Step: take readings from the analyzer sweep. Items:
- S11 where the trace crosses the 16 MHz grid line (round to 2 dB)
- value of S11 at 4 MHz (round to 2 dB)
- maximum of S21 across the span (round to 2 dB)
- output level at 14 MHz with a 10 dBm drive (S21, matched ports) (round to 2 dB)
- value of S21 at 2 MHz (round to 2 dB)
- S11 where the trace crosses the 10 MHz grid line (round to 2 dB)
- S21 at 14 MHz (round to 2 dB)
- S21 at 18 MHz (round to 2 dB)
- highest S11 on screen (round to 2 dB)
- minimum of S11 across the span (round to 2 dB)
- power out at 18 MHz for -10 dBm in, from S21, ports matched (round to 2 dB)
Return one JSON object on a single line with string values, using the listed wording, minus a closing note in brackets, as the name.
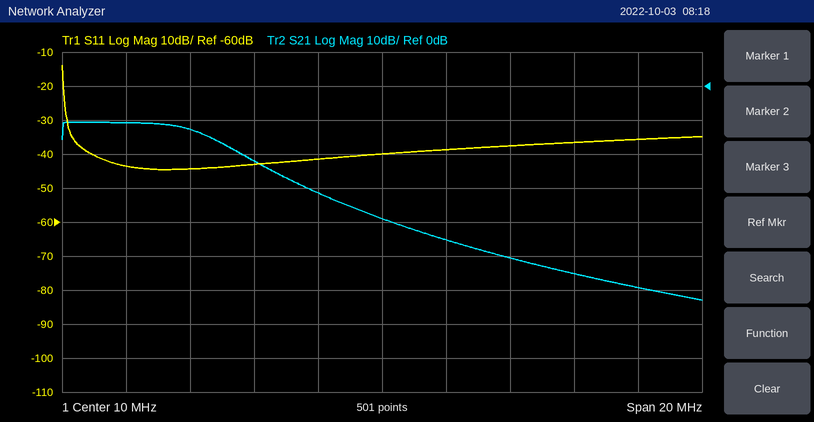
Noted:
{"S11 where the trace crosses the 16 MHz grid line": "-36 dB", "value of S11 at 4 MHz": "-44 dB", "maximum of S21 across the span": "-10 dB", "output level at 14 MHz with a 10 dBm drive (S21, matched ports)": "-40 dBm", "value of S21 at 2 MHz": "-10 dB", "S11 where the trace crosses the 10 MHz grid line": "-40 dB", "S21 at 14 MHz": "-50 dB", "S21 at 18 MHz": "-60 dB", "highest S11 on screen": "-14 dB", "minimum of S11 across the span": "-44 dB", "power out at 18 MHz for -10 dBm in, from S21, ports matched": "-70 dBm"}
